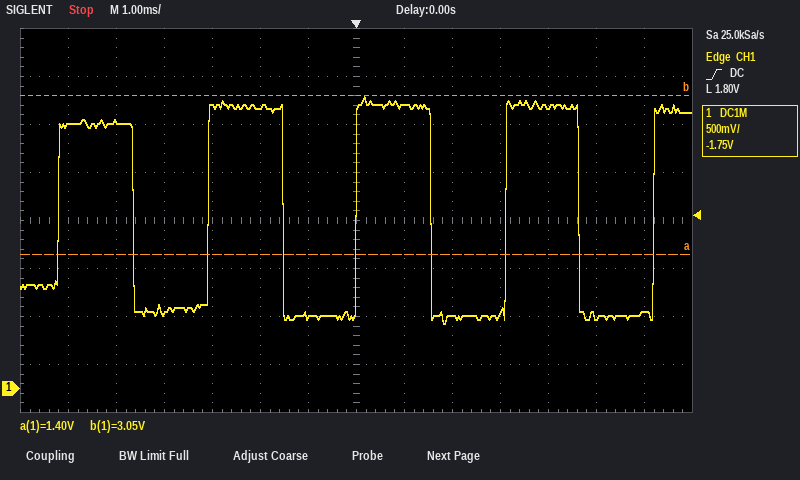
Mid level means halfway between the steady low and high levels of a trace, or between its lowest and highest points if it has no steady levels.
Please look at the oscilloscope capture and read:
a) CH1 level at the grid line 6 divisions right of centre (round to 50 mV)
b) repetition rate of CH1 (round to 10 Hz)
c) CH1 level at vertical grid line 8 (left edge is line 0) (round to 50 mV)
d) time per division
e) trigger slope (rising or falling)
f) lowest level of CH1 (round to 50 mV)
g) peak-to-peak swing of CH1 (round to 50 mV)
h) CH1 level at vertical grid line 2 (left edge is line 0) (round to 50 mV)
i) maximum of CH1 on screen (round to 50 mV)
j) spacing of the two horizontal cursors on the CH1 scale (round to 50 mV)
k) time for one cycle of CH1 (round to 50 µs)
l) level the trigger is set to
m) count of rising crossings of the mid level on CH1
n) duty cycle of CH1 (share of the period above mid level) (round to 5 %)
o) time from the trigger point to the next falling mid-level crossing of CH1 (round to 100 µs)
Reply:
800 mV
320 Hz
2.95 V
1 ms
rising
700 mV
2.35 V
2.80 V
3.05 V
1.65 V
3.10 ms
1.80 V
5
50 %
1.6 ms
